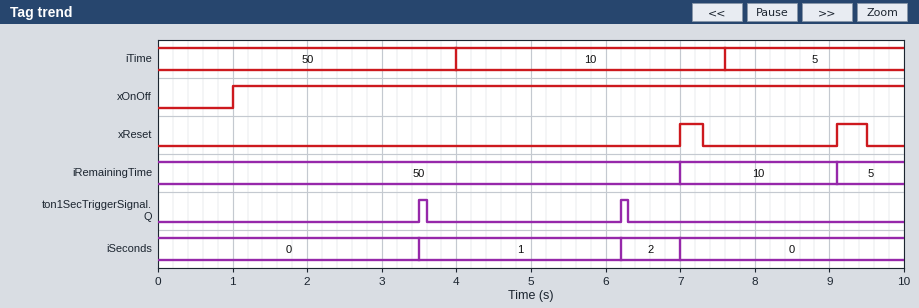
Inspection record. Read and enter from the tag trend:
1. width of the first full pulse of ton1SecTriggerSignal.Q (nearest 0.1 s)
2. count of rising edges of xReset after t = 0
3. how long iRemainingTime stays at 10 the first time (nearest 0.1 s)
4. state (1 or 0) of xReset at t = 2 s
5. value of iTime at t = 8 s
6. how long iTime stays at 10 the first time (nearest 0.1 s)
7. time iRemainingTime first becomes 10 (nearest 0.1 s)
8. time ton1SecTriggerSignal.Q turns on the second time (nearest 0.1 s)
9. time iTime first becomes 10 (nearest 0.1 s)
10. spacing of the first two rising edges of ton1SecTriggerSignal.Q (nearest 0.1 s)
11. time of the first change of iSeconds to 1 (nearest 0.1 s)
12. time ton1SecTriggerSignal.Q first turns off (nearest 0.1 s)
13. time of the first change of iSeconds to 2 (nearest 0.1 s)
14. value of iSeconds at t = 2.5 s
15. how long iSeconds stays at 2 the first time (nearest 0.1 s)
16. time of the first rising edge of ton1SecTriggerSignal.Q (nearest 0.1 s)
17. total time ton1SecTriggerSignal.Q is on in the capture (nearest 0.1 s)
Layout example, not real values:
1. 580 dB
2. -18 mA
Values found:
1. 0.1 s
2. 2
3. 2.1 s
4. 0
5. 5
6. 3.6 s
7. 7.0 s
8. 6.2 s
9. 4.0 s
10. 2.7 s
11. 3.5 s
12. 3.6 s
13. 6.2 s
14. 0
15. 0.8 s
16. 3.5 s
17. 0.2 s
